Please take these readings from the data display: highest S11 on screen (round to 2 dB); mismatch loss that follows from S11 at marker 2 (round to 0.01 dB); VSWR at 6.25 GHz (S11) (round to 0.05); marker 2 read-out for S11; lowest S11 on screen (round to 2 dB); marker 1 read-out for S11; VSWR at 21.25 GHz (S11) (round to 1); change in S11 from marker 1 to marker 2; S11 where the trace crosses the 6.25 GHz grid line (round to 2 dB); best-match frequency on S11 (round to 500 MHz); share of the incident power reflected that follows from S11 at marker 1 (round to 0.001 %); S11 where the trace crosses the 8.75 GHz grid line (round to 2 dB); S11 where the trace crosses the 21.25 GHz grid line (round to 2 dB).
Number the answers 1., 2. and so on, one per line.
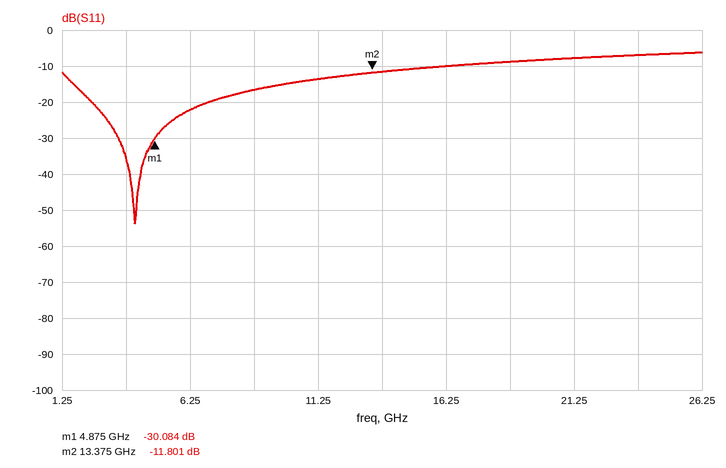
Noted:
1. -6 dB
2. 0.30 dB
3. 1.15
4. -11.801 dB
5. -54 dB
6. -30.084 dB
7. 2
8. 18.283 dB
9. -22 dB
10. 4.0 GHz
11. 0.098 %
12. -16 dB
13. -8 dB
